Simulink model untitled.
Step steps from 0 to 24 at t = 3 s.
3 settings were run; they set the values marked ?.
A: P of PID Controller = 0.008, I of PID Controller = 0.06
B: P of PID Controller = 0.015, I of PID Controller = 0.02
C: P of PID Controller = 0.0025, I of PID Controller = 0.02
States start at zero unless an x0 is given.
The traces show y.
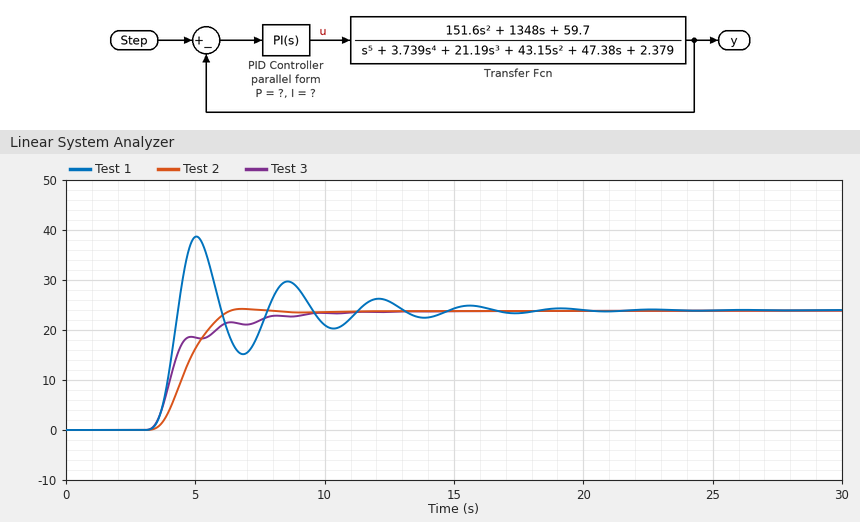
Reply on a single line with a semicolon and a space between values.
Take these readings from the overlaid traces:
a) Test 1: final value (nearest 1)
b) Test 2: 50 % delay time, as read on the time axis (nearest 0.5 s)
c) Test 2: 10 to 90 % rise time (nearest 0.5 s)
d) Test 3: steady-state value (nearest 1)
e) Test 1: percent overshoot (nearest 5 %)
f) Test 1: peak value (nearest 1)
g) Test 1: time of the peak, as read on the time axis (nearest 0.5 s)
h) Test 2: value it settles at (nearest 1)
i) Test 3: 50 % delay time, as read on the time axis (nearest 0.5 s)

24; 4.5 s; 2.0 s; 24; 60 %; 39; 5.0 s; 24; 4.0 s
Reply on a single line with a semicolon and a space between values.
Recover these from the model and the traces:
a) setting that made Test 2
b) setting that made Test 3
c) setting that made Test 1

C; B; A
